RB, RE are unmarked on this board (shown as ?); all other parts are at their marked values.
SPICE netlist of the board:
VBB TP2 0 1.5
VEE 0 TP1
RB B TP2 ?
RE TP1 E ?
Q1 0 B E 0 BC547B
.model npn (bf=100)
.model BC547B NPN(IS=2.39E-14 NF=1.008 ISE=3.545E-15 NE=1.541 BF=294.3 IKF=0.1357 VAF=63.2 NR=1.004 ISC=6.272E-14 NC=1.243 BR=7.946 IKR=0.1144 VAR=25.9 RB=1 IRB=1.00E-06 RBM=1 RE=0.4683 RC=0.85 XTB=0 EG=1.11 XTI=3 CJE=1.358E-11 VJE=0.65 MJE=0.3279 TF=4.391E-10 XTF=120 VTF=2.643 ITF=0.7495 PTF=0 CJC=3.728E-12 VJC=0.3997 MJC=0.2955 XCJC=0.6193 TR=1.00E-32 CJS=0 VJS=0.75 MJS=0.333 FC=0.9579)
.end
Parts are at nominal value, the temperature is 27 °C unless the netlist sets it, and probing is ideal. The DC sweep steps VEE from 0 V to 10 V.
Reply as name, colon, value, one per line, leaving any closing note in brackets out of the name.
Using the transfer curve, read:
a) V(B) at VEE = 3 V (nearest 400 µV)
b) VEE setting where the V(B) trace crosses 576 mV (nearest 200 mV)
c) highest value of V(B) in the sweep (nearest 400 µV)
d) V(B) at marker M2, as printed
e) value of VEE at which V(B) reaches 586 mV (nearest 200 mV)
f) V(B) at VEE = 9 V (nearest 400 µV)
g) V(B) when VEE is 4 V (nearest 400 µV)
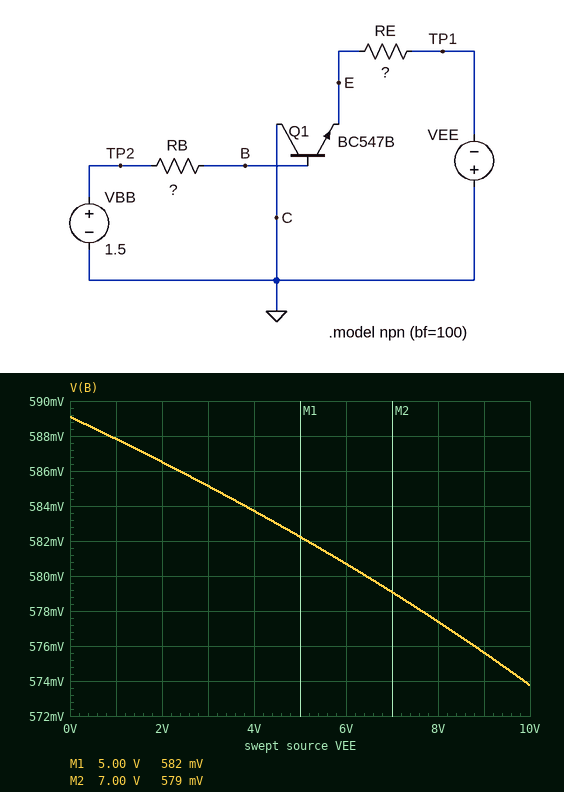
V(B) at VEE = 3 V: 585.2 mV
VEE setting where the V(B) trace crosses 576 mV: 8.8 V
highest value of V(B) in the sweep: 589.2 mV
V(B) at marker M2, as printed: 579 mV
value of VEE at which V(B) reaches 586 mV: 2.4 V
V(B) at VEE = 9 V: 575.6 mV
V(B) when VEE is 4 V: 583.6 mV
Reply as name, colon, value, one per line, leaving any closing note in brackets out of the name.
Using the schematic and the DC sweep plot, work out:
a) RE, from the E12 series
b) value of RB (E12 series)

RE, from the E12 series: 3.3 kΩ
value of RB: 33 kΩ
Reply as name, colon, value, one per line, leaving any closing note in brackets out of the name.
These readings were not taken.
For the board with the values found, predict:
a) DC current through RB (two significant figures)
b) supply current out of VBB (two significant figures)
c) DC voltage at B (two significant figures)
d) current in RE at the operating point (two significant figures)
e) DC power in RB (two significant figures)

DC current through RB: 28 µA
supply current out of VBB: 28 µA
DC voltage at B: 590 mV
current in RE at the operating point: 640 nA
DC power in RB: 25 µW
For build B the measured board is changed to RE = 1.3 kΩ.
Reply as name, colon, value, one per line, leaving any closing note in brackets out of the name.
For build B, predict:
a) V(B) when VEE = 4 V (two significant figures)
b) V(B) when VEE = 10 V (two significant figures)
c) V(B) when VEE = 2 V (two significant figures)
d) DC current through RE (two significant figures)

V(B) when VEE = 4 V: 570 mV
V(B) when VEE = 10 V: 510 mV
V(B) when VEE = 2 V: 580 mV
DC current through RE: 1.5 µA
